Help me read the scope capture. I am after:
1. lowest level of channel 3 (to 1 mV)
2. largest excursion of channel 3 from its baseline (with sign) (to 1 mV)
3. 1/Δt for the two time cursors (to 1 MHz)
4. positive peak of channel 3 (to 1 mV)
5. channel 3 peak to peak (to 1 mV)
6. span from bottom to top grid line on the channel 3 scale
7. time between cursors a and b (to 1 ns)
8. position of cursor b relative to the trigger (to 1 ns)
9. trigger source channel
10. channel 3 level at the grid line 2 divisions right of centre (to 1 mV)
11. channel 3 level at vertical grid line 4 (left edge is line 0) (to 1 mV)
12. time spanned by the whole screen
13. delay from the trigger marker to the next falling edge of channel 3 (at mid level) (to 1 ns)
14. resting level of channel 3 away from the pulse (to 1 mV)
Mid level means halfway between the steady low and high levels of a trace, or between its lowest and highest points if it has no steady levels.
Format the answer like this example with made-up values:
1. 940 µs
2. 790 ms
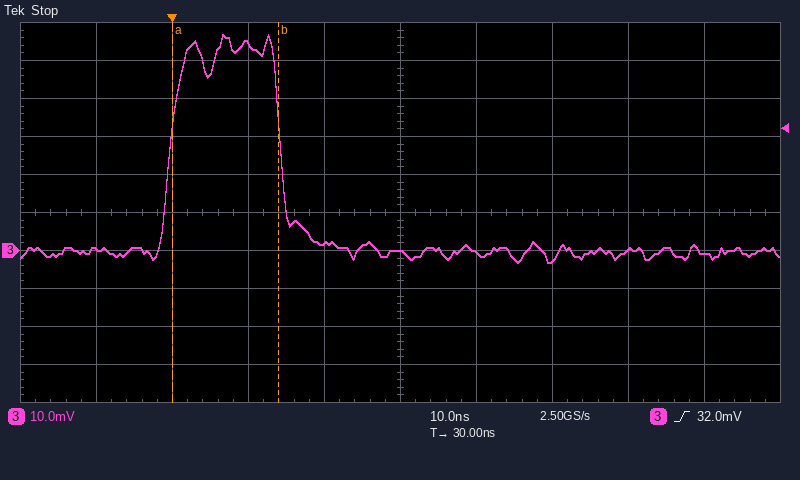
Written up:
1. -3 mV
2. +57 mV
3. 71 MHz
4. 57 mV
5. 60 mV
6. 100 mV
7. 14 ns
8. +14 ns
9. channel 3
10. -2 mV
11. 2 mV
12. 100 ns
13. 14 ns
14. 0 mV
